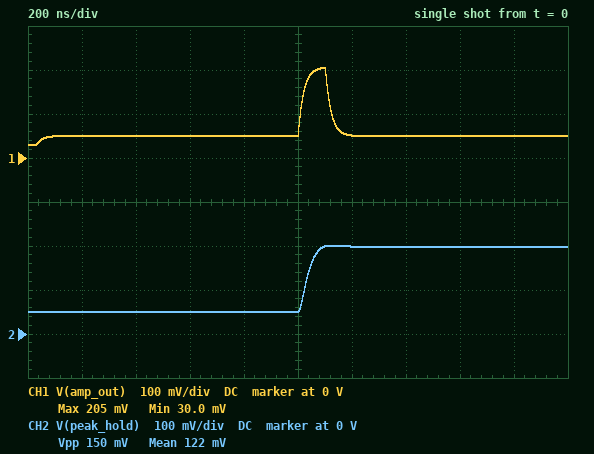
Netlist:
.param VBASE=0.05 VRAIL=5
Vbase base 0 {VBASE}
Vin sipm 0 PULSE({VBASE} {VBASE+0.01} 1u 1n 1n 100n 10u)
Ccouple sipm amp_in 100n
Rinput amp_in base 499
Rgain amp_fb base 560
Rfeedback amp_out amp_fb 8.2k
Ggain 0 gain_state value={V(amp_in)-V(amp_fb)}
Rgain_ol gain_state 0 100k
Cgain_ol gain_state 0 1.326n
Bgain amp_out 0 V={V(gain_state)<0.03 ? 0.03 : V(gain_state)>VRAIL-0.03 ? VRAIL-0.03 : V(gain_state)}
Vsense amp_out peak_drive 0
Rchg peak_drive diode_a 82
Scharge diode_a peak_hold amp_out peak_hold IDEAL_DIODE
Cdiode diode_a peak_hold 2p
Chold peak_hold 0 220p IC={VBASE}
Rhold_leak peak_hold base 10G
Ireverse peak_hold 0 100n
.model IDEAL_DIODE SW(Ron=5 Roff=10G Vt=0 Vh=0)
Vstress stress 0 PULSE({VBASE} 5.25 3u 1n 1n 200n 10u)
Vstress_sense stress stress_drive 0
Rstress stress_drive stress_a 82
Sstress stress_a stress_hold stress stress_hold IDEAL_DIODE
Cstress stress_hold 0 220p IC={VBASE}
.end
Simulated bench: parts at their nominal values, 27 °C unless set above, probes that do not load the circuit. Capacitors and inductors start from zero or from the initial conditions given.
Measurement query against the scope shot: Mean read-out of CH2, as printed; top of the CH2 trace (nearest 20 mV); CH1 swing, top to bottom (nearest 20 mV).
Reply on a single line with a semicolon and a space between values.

122 mV; 200 mV; 180 mV
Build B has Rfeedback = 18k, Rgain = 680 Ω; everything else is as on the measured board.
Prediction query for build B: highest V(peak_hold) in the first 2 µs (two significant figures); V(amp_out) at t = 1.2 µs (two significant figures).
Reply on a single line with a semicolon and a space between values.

290 mV; 67 mV
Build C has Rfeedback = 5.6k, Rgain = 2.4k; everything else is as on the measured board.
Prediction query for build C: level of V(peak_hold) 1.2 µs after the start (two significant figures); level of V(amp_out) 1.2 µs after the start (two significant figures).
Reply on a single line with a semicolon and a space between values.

83 mV; 50 mV
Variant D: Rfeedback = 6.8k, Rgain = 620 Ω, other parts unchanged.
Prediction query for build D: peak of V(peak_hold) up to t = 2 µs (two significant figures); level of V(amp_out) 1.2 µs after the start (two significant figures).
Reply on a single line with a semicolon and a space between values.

170 mV; 50 mV
